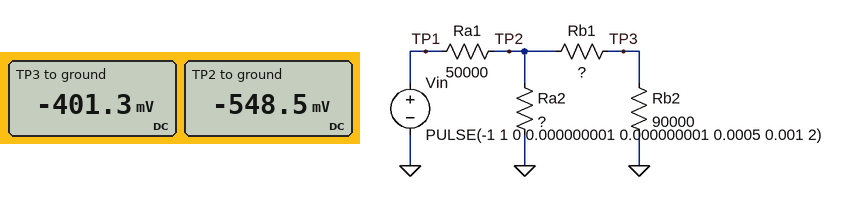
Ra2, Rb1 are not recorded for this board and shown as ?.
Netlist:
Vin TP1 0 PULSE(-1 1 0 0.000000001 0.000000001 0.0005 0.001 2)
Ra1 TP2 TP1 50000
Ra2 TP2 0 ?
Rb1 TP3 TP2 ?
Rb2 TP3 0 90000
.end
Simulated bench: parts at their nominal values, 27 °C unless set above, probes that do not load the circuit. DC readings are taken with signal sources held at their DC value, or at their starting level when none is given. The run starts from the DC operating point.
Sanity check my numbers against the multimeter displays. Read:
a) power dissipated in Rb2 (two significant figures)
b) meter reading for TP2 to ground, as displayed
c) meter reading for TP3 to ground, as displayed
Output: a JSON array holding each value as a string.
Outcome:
["1.8 µW", "-548.5 mV", "-401.3 mV"]
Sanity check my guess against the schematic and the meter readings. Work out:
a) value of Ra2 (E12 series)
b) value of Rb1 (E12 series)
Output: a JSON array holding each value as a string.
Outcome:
["120 kΩ", "33 kΩ"]
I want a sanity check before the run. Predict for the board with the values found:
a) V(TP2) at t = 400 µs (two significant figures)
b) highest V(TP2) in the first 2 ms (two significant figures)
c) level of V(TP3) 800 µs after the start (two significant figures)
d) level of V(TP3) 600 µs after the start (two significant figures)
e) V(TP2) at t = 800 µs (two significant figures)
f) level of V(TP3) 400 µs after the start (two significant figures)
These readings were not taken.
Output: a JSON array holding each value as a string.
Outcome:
["550 mV", "550 mV", "-400 mV", "-400 mV", "-550 mV", "400 mV"]
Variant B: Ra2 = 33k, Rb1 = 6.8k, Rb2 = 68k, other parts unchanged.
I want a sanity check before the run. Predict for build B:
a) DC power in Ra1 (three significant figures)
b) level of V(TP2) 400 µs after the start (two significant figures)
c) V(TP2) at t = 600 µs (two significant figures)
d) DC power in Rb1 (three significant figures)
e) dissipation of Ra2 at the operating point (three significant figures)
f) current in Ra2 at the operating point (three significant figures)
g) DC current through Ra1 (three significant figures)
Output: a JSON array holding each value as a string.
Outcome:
["9.41 µW", "310 mV", "-310 mV", "120 nW", "2.99 µW", "9.52 µA", "13.7 µA"]
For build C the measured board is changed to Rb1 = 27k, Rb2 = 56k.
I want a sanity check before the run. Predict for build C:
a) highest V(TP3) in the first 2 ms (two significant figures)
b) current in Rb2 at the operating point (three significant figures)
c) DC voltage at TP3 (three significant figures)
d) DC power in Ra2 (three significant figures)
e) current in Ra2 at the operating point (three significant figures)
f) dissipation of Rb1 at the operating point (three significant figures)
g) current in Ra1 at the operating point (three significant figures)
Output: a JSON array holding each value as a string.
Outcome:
["330 mV", "5.97 µA", "-334 mV", "2.04 µW", "4.13 µA", "961 nW", "10.1 µA"]
